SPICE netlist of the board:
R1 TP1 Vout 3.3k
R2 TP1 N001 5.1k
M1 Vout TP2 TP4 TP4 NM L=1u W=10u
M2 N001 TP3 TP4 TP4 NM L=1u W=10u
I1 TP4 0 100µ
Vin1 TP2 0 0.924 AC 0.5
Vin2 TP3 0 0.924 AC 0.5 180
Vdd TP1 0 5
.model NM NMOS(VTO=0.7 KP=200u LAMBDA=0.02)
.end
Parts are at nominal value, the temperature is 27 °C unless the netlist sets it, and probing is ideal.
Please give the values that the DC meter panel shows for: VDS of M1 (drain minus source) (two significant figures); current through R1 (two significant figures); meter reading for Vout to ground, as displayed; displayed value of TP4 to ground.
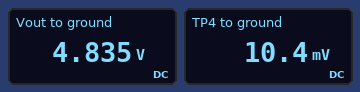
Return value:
4.8 V
50 µA
4.835 V
10.4 mV
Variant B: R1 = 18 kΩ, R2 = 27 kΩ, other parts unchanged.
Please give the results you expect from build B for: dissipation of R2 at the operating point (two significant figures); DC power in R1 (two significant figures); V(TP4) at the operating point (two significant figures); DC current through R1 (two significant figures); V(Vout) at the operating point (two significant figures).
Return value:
67 µW
45 µW
8.6 mV
50 µA
4.1 V
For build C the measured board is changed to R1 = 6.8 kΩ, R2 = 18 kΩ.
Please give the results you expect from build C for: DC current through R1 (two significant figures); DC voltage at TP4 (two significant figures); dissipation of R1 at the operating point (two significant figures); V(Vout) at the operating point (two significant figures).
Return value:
50 µA
9.6 mV
17 µW
4.7 V
